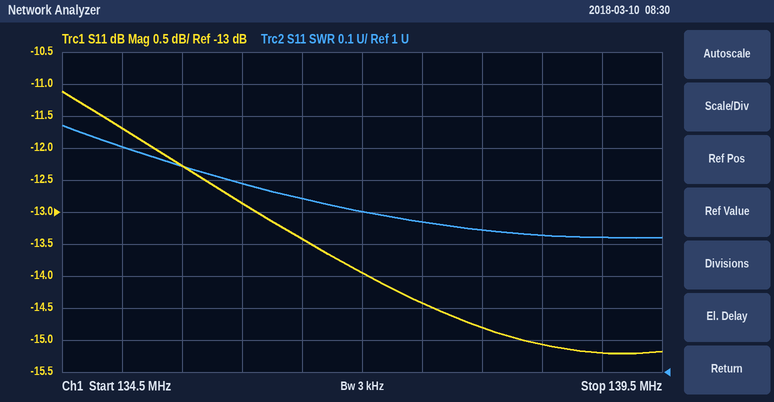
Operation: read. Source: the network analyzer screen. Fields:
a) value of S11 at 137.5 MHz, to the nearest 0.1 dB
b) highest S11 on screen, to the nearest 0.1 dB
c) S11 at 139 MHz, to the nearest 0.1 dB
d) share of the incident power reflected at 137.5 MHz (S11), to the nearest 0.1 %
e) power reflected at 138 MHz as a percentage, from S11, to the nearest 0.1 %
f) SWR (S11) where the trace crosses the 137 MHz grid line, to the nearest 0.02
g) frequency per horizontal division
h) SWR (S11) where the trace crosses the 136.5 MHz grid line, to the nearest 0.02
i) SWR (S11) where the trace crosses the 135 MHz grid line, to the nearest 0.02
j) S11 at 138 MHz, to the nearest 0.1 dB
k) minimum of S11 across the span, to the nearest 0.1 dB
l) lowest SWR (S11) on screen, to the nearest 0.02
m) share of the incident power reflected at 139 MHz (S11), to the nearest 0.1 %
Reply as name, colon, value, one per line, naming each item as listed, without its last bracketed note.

value of S11 at 137.5 MHz, to the nearest 0.1 dB: -14.4 dB
highest S11 on screen, to the nearest 0.1 dB: -11.1 dB
S11 at 139 MHz, to the nearest 0.1 dB: -15.2 dB
share of the incident power reflected at 137.5 MHz (S11), to the nearest 0.1 %: 3.6 %
power reflected at 138 MHz as a percentage, from S11, to the nearest 0.1 %: 3.3 %
SWR (S11) where the trace crosses the 137 MHz grid line, to the nearest 0.02: 1.50
frequency per horizontal division: 500 kHz
SWR (S11) where the trace crosses the 136.5 MHz grid line, to the nearest 0.02: 1.54
SWR (S11) where the trace crosses the 135 MHz grid line, to the nearest 0.02: 1.70
S11 at 138 MHz, to the nearest 0.1 dB: -14.8 dB
minimum of S11 across the span, to the nearest 0.1 dB: -15.2 dB
lowest SWR (S11) on screen, to the nearest 0.02: 1.42
share of the incident power reflected at 139 MHz (S11), to the nearest 0.1 %: 3.0 %
